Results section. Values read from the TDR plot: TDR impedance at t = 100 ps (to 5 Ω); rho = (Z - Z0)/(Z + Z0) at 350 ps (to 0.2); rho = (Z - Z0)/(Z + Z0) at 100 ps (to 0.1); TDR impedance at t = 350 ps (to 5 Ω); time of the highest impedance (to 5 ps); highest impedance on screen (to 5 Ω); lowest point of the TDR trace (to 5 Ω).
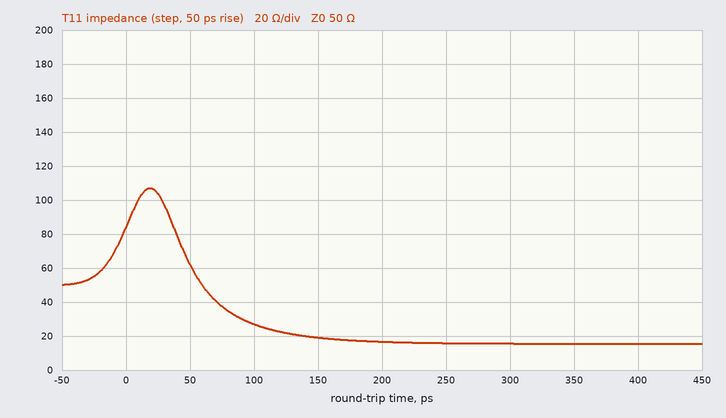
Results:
25 Ω
-0.6
-0.3
15 Ω
20 ps
105 Ω
15 Ω
